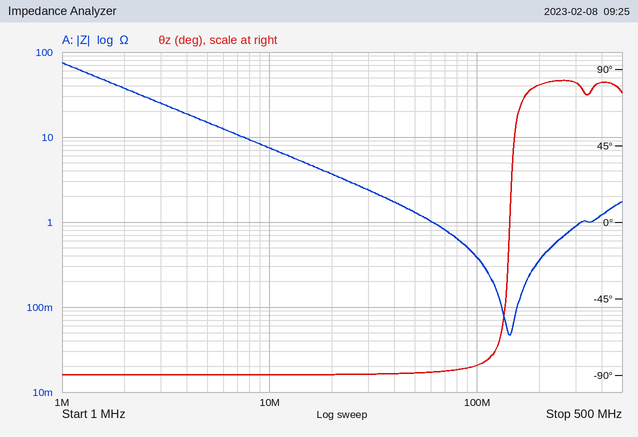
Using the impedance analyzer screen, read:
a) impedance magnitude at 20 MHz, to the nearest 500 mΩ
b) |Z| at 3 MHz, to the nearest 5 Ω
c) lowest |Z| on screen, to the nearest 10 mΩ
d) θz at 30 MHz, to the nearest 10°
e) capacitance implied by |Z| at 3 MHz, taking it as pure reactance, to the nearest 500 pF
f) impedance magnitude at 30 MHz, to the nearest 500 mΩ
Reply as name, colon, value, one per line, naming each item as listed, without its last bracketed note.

impedance magnitude at 20 MHz, to the nearest 500 mΩ: 3.5 Ω
|Z| at 3 MHz, to the nearest 5 Ω: 25 Ω
lowest |Z| on screen, to the nearest 10 mΩ: 50 mΩ
θz at 30 MHz, to the nearest 10°: -90°
capacitance implied by |Z| at 3 MHz, taking it as pure reactance, to the nearest 500 pF: 2.0 nF
impedance magnitude at 30 MHz, to the nearest 500 mΩ: 2.5 Ω
